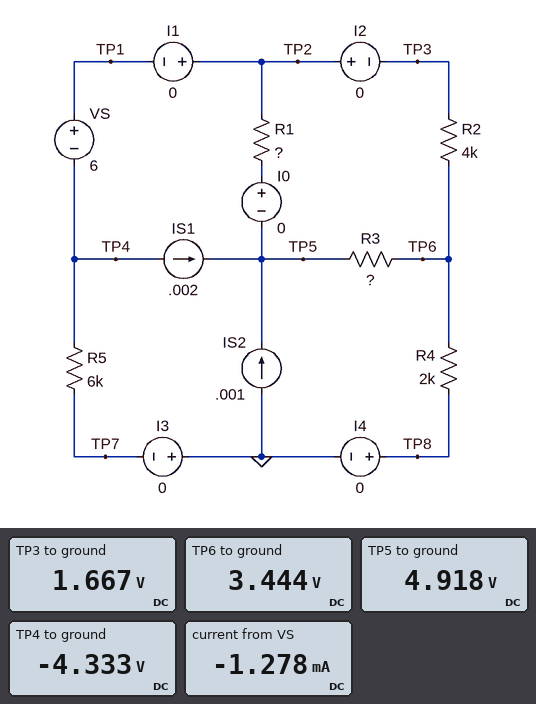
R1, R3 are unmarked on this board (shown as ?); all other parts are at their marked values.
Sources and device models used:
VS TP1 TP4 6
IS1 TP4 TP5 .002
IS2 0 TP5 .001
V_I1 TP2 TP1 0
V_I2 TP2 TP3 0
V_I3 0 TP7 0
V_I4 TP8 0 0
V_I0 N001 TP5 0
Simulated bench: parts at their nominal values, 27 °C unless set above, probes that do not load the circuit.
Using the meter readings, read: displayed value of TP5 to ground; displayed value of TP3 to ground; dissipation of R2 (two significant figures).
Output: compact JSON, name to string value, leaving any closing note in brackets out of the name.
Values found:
{"displayed value of TP5 to ground": "4.918 V", "displayed value of TP3 to ground": "1.667 V", "dissipation of R2": "790 µW"}
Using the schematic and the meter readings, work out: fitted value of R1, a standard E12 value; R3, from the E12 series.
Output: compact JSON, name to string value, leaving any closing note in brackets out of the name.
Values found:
{"fitted value of R1, a standard E12 value": "3.9 kΩ", "R3, from the E12 series": "680 Ω"}
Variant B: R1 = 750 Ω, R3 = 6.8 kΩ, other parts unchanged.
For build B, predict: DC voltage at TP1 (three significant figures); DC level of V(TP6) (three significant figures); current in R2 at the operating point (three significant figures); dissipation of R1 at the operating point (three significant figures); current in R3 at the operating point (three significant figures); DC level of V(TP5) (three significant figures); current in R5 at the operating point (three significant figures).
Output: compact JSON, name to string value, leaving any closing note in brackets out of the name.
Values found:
{"DC voltage at TP1": "4.78 V", "DC level of V(TP6)": "2.41 V", "current in R2 at the operating point": "592 µA", "dissipation of R1 at the operating point": "4.28 mW", "current in R3 at the operating point": "612 µA", "DC level of V(TP5)": "6.57 V", "current in R5 at the operating point": "204 µA"}
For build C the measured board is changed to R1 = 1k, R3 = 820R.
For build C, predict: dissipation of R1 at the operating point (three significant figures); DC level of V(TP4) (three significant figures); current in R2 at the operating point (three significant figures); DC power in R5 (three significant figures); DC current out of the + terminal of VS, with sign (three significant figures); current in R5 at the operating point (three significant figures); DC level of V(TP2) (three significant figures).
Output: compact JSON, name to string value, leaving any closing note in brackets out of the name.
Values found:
{"dissipation of R1 at the operating point": "2.07 mW", "DC level of V(TP4)": "-3.12 V", "current in R2 at the operating point": "40.1 µA", "DC power in R5": "1.62 mW", "DC current out of the + terminal of VS, with sign": "-1.48 mA", "current in R5 at the operating point": "520 µA", "DC level of V(TP2)": "2.88 V"}
